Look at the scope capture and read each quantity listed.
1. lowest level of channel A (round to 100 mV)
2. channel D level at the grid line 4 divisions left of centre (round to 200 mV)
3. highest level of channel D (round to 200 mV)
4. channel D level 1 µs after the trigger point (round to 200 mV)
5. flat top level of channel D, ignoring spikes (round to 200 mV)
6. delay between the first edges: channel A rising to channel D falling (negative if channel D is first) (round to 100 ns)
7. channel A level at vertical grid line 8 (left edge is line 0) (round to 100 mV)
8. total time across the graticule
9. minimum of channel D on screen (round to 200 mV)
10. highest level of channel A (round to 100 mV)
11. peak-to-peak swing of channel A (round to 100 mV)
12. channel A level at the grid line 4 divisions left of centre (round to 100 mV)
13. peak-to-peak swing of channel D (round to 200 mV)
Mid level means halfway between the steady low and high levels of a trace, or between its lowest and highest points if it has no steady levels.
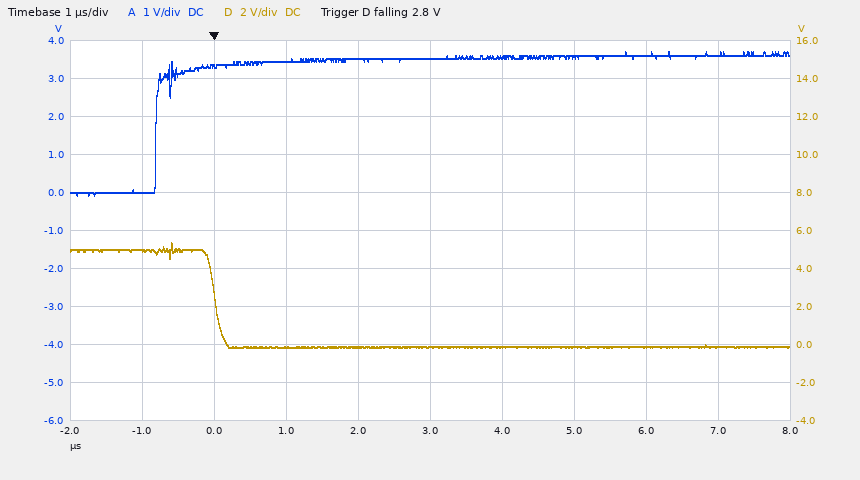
-100 mV
5.0 V
5.4 V
-200 mV
5.0 V
+800 ns
3.6 V
10 µs
-200 mV
3.7 V
3.8 V
0.0 V
5.6 V
